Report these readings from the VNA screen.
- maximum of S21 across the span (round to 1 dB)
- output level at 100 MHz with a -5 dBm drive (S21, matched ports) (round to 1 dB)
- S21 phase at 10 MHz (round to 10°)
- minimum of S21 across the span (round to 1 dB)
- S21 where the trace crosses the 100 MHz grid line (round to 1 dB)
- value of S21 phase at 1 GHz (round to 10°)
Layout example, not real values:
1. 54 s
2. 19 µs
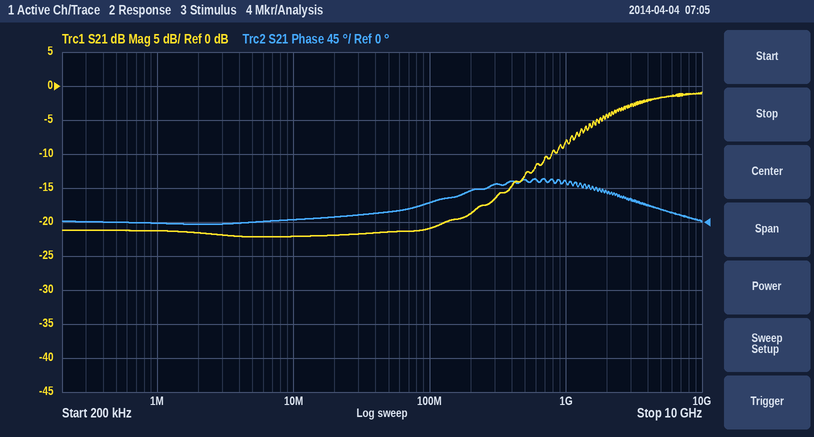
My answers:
1. -1 dB
2. -26 dBm
3. 0°
4. -22 dB
5. -21 dB
6. 50°
